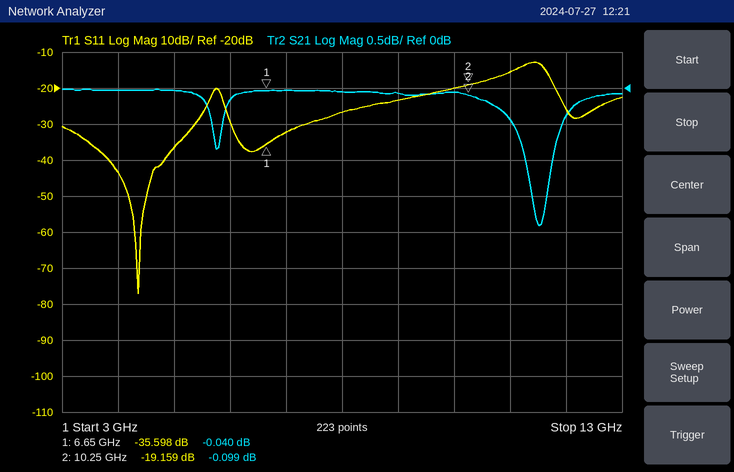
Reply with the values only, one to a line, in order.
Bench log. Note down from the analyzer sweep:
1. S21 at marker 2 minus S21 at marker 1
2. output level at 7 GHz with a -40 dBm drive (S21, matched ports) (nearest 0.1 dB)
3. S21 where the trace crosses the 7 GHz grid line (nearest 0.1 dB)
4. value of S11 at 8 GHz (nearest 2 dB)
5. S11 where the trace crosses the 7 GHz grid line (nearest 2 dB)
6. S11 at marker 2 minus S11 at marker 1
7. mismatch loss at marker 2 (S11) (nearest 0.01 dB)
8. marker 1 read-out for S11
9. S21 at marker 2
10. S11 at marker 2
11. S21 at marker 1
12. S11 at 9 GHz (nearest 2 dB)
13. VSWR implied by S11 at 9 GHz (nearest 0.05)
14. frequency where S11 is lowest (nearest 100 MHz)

-0.059 dB
-40.0 dBm
0.0 dB
-26 dB
-32 dB
16.439 dB
0.05 dB
-35.598 dB
-0.099 dB
-19.159 dB
-0.040 dB
-24 dB
1.15
4.4 GHz
